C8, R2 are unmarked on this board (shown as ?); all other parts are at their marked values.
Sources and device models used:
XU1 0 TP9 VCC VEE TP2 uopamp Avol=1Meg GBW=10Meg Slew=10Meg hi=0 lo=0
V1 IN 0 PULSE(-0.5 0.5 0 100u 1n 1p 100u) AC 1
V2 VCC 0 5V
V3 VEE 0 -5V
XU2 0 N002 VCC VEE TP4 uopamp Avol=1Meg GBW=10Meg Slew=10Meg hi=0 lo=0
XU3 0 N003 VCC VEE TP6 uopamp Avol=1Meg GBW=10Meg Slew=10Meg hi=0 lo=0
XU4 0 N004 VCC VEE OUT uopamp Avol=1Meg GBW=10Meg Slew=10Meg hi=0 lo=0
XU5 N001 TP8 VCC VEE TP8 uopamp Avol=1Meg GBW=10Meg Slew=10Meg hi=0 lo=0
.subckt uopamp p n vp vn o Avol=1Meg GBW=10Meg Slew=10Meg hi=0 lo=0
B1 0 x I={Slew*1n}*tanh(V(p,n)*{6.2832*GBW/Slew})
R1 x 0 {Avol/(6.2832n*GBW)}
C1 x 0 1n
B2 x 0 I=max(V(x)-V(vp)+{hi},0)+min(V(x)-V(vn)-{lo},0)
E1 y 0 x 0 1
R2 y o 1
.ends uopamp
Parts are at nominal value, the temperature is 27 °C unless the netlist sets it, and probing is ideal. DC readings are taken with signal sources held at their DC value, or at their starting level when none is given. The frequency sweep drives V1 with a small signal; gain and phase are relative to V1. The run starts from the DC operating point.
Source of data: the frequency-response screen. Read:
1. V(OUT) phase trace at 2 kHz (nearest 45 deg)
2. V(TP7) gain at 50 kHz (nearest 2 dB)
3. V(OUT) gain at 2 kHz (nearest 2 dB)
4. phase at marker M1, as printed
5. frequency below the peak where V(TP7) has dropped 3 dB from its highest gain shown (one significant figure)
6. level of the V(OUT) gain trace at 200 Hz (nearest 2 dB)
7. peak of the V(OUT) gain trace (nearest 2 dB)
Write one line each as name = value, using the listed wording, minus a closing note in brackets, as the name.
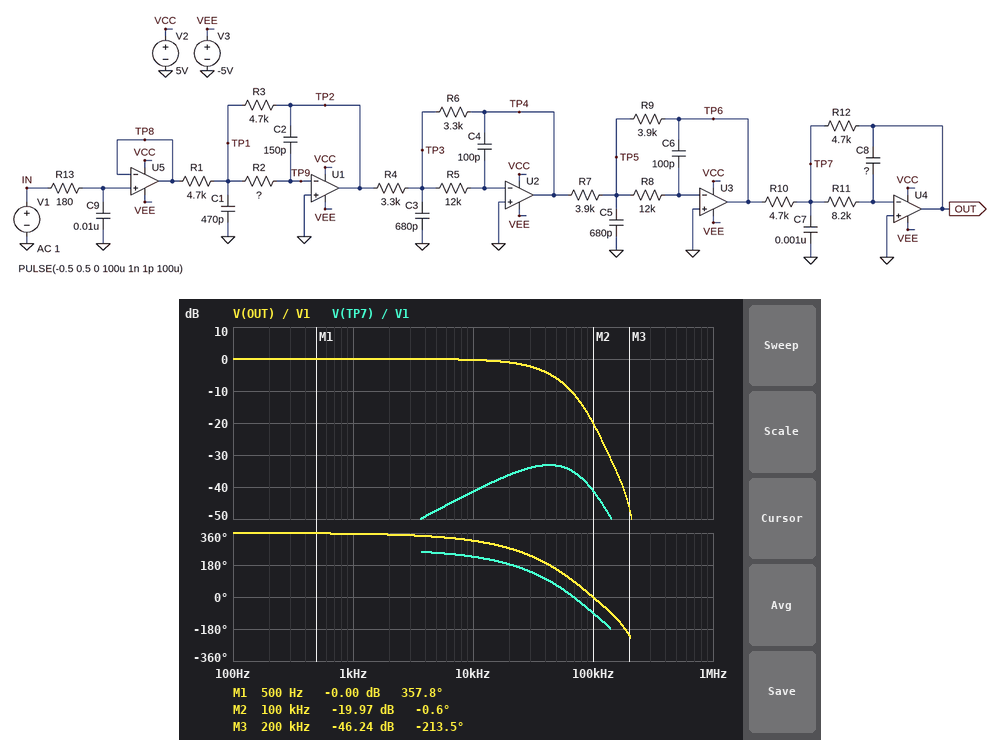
V(OUT) phase trace at 2 kHz = 360 deg
V(TP7) gain at 50 kHz = -34 dB
V(OUT) gain at 2 kHz = 0 dB
phase at marker M1, as printed = 357.8 deg
frequency below the peak where V(TP7) has dropped 3 dB from its highest gain shown = 20 kHz
level of the V(OUT) gain trace at 200 Hz = 0 dB
peak of the V(OUT) gain trace = 0 dB
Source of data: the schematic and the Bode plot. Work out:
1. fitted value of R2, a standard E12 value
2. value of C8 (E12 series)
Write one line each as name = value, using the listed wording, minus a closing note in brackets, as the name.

fitted value of R2, a standard E12 value = 12 kΩ
value of C8 = 15 pF
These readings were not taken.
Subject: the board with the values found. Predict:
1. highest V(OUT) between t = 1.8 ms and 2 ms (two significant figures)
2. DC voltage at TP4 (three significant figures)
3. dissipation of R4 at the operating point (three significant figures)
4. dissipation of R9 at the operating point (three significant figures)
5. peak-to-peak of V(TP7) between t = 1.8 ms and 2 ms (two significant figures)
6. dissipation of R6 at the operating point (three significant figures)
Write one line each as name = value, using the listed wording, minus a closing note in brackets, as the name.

highest V(OUT) between t = 1.8 ms and 2 ms = 420 mV
DC voltage at TP4 = -500 mV
dissipation of R4 at the operating point = 75.8 µW
dissipation of R9 at the operating point = 64.1 µW
peak-to-peak of V(TP7) between t = 1.8 ms and 2 ms = 15 mV
dissipation of R6 at the operating point = 75.8 µW
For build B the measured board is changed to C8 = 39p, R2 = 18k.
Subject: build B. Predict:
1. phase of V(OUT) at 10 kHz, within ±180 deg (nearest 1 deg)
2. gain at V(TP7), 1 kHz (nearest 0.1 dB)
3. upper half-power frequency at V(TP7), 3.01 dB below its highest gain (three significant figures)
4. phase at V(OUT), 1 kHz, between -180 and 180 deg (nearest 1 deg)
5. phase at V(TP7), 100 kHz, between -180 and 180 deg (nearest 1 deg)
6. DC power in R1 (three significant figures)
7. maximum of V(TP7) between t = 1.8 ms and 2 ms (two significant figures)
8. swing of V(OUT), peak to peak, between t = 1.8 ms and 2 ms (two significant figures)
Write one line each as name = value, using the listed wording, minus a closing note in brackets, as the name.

phase of V(OUT) at 10 kHz, within ±180 deg = -51 deg
gain at V(TP7), 1 kHz = -53.5 dB
upper half-power frequency at V(TP7), 3.01 dB below its highest gain = 73.1 kHz
phase at V(OUT), 1 kHz, between -180 and 180 deg = -5 deg
phase at V(TP7), 100 kHz, between -180 and 180 deg = -136 deg
DC power in R1 = 53.2 µW
maximum of V(TP7) between t = 1.8 ms and 2 ms = 28 mV
swing of V(OUT), peak to peak, between t = 1.8 ms and 2 ms = 750 mV
